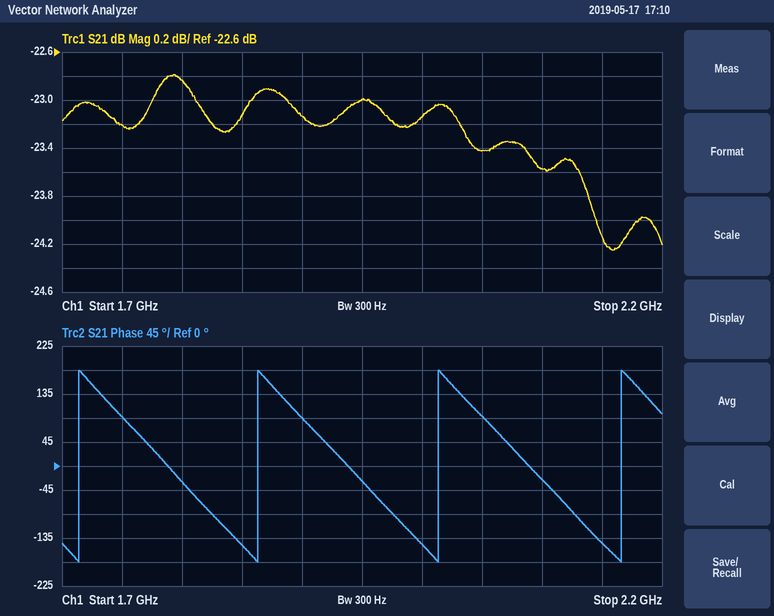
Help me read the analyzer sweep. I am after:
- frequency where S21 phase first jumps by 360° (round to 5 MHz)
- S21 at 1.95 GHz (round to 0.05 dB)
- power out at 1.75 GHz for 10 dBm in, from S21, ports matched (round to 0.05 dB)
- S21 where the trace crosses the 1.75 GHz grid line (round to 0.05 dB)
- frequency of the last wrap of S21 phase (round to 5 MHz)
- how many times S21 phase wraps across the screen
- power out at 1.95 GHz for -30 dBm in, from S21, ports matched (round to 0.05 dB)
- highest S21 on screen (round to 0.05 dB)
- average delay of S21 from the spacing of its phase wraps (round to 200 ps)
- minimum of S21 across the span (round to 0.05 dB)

1.715 GHz
-23.00 dB
-13.20 dBm
-23.20 dB
2.165 GHz
4
-53.00 dBm
-22.80 dB
6.6 ns
-24.25 dB
